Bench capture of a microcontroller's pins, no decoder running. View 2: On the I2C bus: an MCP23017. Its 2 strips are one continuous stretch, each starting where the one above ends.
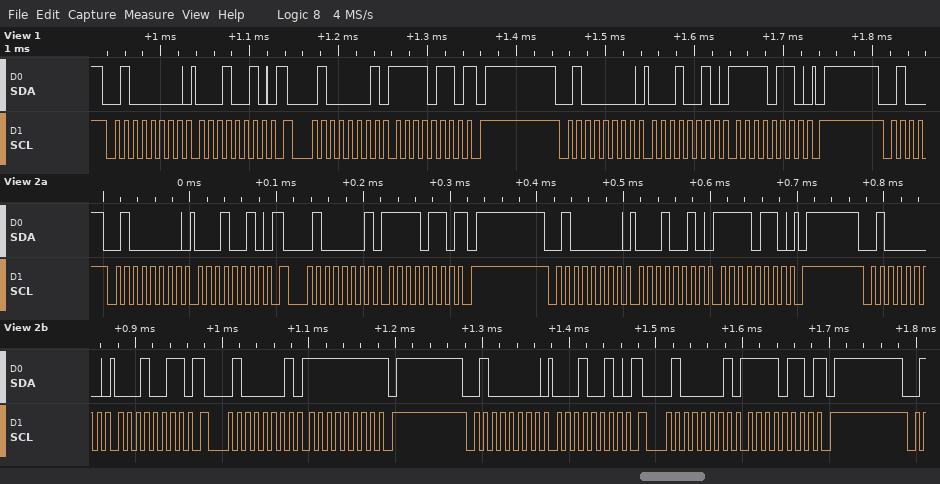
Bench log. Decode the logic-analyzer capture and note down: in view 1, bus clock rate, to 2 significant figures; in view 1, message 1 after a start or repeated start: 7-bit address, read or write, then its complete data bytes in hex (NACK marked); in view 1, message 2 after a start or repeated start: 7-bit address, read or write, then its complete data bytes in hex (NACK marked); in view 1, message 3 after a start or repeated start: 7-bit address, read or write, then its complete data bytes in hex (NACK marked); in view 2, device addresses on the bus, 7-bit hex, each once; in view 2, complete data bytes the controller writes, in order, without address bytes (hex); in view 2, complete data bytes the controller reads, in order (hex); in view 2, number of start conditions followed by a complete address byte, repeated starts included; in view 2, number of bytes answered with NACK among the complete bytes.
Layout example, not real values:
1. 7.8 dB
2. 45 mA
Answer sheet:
1. 100 kHz
2. 0x20 write: 12
3. 0x20 read: F6 NACK
4. 0x20 write: 12 F6
5. 0x20
6. 12 12 F6 13 12
7. F6 FF F6
8. 7
9. 3
